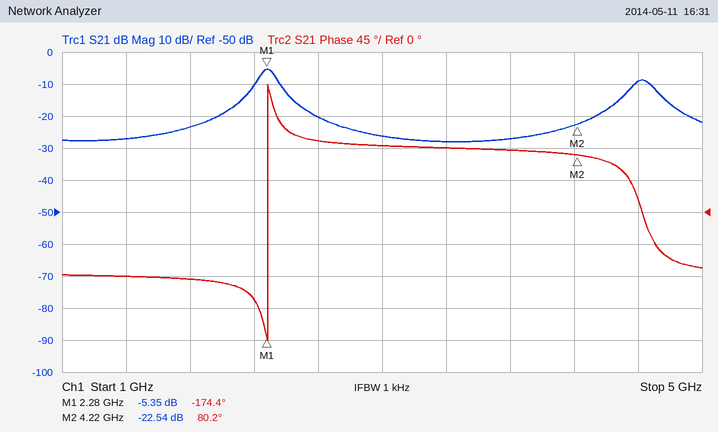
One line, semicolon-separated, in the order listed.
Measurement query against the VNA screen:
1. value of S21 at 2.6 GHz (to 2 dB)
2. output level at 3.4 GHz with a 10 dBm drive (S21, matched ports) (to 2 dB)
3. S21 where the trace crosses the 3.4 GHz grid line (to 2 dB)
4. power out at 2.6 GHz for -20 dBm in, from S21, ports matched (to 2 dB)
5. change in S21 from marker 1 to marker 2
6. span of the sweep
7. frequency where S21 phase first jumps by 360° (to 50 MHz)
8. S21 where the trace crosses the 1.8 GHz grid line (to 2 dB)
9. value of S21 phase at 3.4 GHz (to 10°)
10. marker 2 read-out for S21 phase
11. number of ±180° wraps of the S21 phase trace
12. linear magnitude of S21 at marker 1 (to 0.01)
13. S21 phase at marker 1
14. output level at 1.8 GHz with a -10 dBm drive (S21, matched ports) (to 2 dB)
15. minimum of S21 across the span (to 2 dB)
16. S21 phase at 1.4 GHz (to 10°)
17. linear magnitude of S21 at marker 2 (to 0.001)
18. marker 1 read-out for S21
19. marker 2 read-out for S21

-20 dB; -18 dBm; -28 dB; -40 dBm; -17.19 dB; 4 GHz; 2.30 GHz; -24 dB; 90°; 80.2°; 1; 0.54; -174.4°; -34 dBm; -28 dB; -90°; 0.075; -5.35 dB; -22.54 dB
